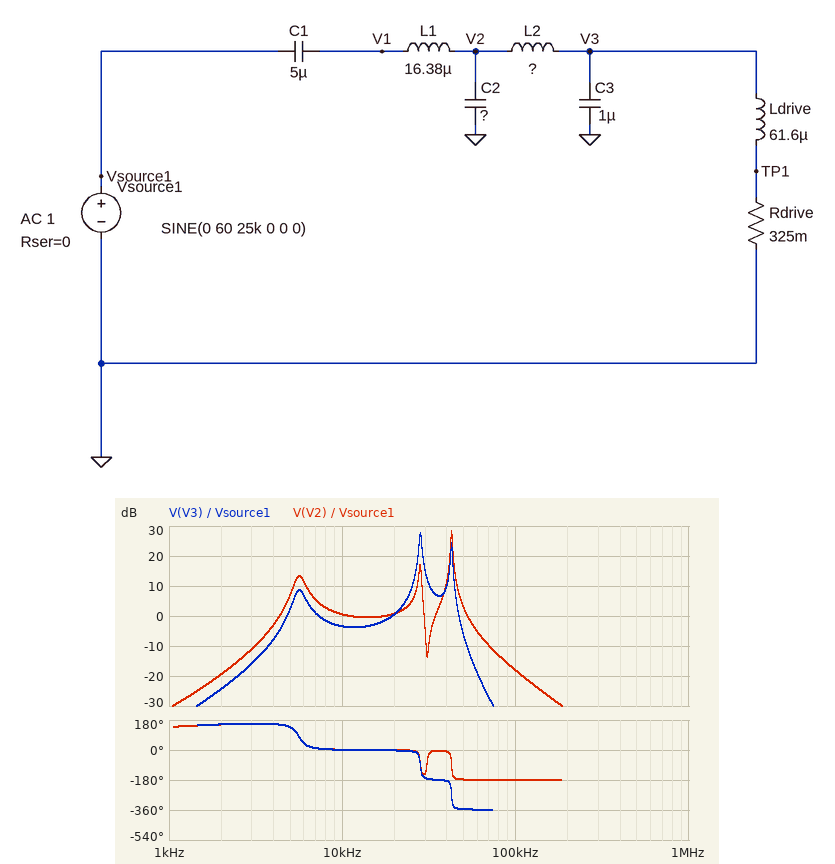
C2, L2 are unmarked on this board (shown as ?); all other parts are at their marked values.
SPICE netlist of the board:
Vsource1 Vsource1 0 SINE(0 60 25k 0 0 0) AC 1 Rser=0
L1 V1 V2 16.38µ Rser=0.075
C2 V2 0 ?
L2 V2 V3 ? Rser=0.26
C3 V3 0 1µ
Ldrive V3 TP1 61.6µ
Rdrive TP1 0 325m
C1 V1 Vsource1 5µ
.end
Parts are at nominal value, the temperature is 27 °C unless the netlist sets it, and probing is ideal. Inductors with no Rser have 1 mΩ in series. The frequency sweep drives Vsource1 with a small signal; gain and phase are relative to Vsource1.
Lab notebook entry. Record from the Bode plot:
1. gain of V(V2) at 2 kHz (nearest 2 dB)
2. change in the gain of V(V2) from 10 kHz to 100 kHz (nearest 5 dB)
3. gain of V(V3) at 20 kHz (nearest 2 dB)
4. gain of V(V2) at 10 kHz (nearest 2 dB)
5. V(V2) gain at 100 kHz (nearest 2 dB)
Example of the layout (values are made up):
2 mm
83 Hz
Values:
-20 dB
-20 dB
0 dB
0 dB
-18 dB
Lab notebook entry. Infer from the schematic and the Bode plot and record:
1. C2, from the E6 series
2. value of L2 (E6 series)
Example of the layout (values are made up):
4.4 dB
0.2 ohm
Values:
1.5 µF
47 µH
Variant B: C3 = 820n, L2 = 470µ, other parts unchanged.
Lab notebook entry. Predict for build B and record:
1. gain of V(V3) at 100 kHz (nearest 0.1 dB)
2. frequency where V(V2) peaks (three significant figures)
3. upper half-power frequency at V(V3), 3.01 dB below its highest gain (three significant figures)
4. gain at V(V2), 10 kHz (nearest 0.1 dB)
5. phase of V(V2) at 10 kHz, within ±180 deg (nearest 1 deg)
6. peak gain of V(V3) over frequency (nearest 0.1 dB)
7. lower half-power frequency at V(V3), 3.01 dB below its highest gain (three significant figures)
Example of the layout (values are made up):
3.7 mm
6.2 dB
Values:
-61.6 dB
37.0 kHz
24.2 kHz
-1.1 dB
0 deg
13.5 dB
23.4 kHz
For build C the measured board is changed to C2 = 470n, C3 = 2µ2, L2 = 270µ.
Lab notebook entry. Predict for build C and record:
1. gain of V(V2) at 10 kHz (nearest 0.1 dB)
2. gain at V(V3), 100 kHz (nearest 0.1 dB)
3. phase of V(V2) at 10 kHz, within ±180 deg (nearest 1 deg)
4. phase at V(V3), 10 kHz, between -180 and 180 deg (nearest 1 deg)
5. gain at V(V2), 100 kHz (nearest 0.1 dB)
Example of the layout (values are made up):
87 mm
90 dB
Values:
0.2 dB
-52.7 dB
0 deg
-6 deg
-5.5 dB
